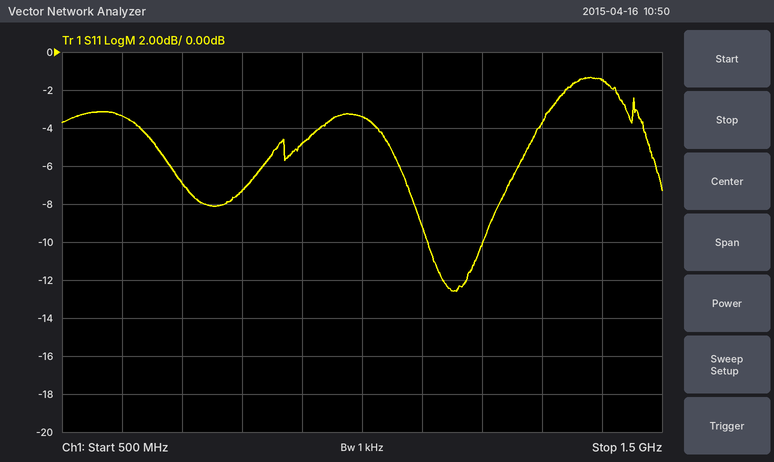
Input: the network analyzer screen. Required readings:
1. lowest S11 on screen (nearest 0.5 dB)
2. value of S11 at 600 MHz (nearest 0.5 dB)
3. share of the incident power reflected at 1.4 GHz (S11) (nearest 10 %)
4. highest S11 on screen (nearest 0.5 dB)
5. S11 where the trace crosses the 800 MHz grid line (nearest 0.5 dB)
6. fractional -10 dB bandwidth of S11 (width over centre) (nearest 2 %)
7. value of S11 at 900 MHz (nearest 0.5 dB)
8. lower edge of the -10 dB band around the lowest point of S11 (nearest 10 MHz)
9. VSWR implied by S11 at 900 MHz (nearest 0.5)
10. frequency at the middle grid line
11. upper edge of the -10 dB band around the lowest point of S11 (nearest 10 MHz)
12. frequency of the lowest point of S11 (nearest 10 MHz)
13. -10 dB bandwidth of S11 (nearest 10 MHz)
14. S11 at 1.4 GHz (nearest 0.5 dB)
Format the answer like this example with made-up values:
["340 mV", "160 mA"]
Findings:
["-12.5 dB", "-3.5 dB", "70 %", "-1.5 dB", "-7.5 dB", "8 %", "-5.0 dB", "1.11 GHz", "3.5", "1 GHz", "1.20 GHz", "1.15 GHz", "90 MHz", "-1.5 dB"]
